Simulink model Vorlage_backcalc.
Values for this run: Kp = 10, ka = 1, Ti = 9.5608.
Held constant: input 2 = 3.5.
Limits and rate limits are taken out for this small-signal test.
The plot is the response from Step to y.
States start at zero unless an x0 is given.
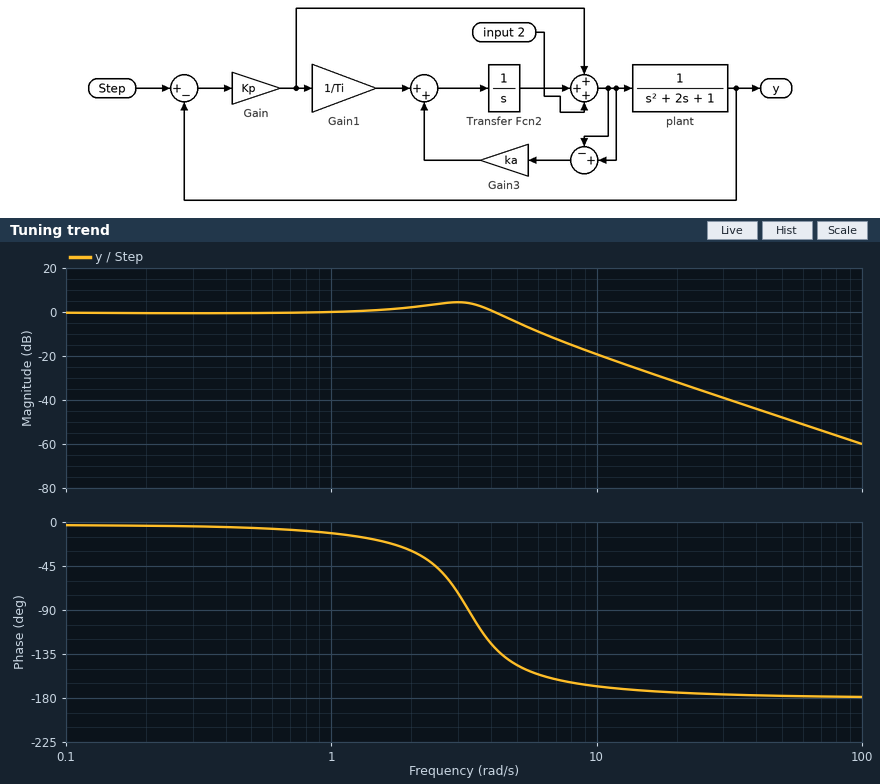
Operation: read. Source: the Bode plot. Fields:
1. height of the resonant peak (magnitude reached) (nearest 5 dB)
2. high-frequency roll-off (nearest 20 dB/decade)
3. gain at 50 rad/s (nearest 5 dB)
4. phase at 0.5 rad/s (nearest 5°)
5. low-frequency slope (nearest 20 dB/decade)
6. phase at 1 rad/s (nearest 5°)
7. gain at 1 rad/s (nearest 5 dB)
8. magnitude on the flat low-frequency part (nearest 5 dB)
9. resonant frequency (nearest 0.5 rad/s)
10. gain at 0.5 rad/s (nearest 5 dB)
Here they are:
5 dB
-40 dB/decade
-50 dB
-5°
0 dB/decade
-10°
0 dB
0 dB
3.0 rad/s
0 dB
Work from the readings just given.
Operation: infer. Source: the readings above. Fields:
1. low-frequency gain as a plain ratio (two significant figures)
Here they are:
1.0
